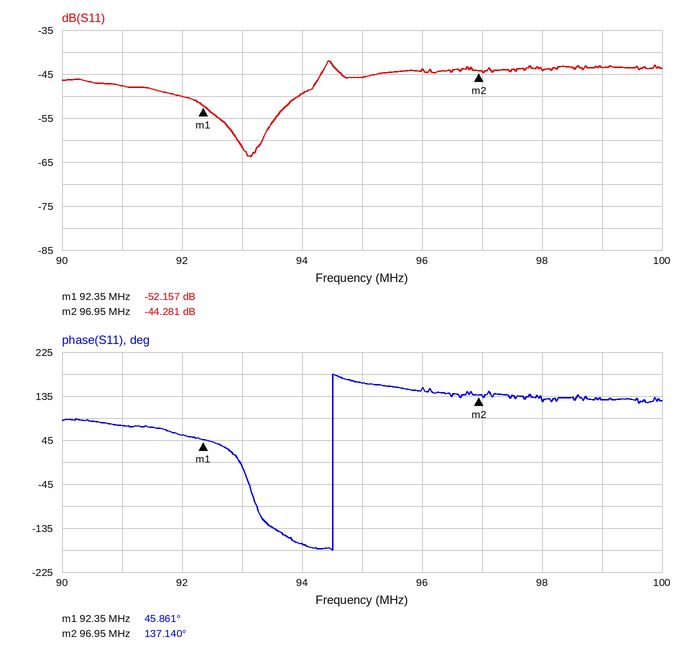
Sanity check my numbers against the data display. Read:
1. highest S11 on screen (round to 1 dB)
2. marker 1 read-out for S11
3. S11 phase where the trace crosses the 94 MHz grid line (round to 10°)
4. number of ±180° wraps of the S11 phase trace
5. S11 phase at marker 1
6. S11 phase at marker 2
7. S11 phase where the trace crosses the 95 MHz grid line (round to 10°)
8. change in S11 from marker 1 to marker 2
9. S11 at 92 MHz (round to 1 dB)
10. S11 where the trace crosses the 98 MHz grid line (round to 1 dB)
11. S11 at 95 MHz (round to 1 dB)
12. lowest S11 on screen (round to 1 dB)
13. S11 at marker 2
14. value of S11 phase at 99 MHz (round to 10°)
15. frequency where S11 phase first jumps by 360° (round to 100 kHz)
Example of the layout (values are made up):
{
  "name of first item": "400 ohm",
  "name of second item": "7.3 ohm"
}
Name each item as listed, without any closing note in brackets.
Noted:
{
  "highest S11 on screen": "-42 dB",
  "marker 1 read-out for S11": "-52.157 dB",
  "S11 phase where the trace crosses the 94 MHz grid line": "-170°",
  "number of ±180° wraps of the S11 phase trace": "1",
  "S11 phase at marker 1": "45.861°",
  "S11 phase at marker 2": "137.140°",
  "S11 phase where the trace crosses the 95 MHz grid line": "160°",
  "change in S11 from marker 1 to marker 2": "7.876 dB",
  "S11 at 92 MHz": "-50 dB",
  "S11 where the trace crosses the 98 MHz grid line": "-44 dB",
  "S11 at 95 MHz": "-46 dB",
  "lowest S11 on screen": "-64 dB",
  "S11 at marker 2": "-44.281 dB",
  "value of S11 phase at 99 MHz": "130°",
  "frequency where S11 phase first jumps by 360°": "94.5 MHz"
}
